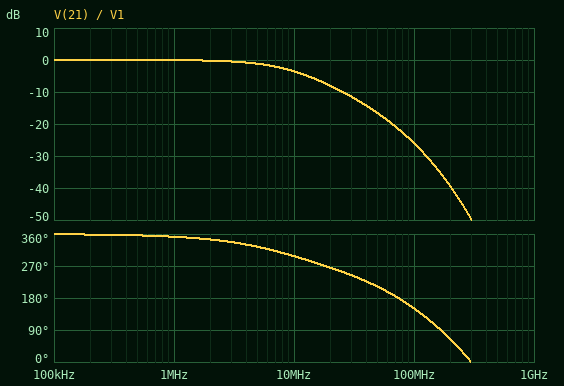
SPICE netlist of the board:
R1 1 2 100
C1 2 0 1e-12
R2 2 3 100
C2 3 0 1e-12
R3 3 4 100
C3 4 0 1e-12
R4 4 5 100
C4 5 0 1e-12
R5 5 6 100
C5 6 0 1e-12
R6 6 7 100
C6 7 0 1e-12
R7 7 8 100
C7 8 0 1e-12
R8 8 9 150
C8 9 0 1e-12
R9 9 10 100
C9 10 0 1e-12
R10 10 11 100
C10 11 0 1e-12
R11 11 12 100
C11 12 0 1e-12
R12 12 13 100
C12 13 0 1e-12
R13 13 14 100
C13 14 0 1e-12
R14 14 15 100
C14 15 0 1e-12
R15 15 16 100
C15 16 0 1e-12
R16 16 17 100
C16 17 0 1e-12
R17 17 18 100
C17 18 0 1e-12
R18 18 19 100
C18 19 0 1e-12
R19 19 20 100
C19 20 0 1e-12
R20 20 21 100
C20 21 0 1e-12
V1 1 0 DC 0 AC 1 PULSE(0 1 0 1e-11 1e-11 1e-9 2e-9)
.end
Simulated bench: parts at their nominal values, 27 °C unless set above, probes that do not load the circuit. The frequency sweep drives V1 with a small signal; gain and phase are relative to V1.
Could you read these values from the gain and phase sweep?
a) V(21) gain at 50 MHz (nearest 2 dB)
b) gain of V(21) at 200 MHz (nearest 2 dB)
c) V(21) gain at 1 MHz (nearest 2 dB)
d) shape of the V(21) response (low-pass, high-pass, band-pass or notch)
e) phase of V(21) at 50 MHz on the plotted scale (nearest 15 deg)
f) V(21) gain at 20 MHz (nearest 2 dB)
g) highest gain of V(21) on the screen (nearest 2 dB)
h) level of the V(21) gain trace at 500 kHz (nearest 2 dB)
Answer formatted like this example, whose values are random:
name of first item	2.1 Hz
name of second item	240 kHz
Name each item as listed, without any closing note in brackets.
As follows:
V(21) gain at 50 MHz	-16 dB
gain of V(21) at 200 MHz	-40 dB
V(21) gain at 1 MHz	0 dB
shape of the V(21) response	low-pass
phase of V(21) at 50 MHz on the plotted scale	210 deg
V(21) gain at 20 MHz	-8 dB
highest gain of V(21) on the screen	0 dB
level of the V(21) gain trace at 500 kHz	0 dB
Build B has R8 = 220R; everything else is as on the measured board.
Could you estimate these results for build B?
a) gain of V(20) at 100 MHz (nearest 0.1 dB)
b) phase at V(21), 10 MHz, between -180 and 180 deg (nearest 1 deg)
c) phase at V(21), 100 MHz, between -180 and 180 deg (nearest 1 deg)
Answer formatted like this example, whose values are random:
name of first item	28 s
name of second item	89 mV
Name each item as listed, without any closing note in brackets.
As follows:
gain of V(20) at 100 MHz	-26.5 dB
phase at V(21), 10 MHz, between -180 and 180 deg	-64 deg
phase at V(21), 100 MHz, between -180 and 180 deg	148 deg
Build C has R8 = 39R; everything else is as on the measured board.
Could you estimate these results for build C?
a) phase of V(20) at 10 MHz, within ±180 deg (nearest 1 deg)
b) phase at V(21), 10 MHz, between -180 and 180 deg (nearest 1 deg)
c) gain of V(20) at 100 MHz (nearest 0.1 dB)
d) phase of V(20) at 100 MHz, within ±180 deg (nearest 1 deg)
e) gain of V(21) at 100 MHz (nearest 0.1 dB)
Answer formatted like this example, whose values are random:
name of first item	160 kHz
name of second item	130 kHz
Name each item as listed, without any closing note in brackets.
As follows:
phase of V(20) at 10 MHz, within ±180 deg	-59 deg
phase at V(21), 10 MHz, between -180 and 180 deg	-60 deg
gain of V(20) at 100 MHz	-25.1 dB
phase of V(20) at 100 MHz, within ±180 deg	159 deg
gain of V(21) at 100 MHz	-25.2 dB
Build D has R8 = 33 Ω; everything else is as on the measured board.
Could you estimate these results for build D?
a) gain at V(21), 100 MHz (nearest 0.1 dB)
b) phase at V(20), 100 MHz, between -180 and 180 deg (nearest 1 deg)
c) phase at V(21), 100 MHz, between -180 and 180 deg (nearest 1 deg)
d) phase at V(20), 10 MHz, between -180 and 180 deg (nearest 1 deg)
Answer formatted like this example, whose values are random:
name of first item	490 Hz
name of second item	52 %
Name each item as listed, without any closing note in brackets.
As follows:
gain at V(21), 100 MHz	-25.1 dB
phase at V(20), 100 MHz, between -180 and 180 deg	160 deg
phase at V(21), 100 MHz, between -180 and 180 deg	156 deg
phase at V(20), 10 MHz, between -180 and 180 deg	-59 deg
